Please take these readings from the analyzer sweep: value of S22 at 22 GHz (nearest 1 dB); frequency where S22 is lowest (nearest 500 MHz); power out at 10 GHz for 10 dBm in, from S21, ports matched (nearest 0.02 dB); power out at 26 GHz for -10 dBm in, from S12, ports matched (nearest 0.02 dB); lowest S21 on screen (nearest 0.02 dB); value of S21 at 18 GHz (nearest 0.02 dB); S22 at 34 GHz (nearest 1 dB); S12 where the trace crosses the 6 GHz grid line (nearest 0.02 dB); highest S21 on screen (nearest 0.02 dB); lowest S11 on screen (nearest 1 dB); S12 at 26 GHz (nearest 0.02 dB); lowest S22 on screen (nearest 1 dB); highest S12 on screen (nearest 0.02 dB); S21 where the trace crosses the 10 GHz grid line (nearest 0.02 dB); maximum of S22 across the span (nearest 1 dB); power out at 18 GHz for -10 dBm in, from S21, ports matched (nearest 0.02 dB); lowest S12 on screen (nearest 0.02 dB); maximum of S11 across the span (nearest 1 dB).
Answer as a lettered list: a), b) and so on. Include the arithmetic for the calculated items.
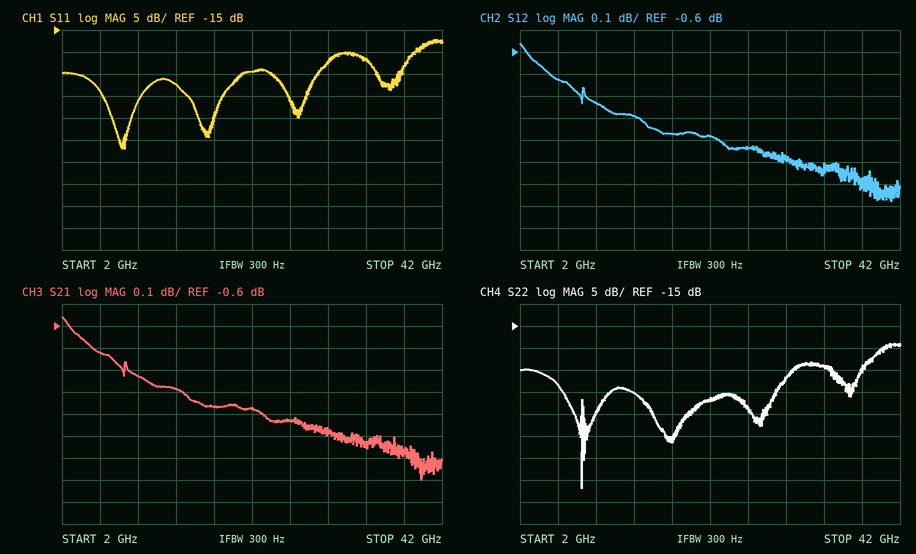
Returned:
a) -32 dB
b) 8.5 GHz
c) 10 dBm + (-0.82 dB) = 9.18 dBm
d) -10 dBm + (-1.04 dB) = -11.04 dBm
e) -1.30 dB
f) -0.96 dB
g) -24 dB
h) -0.72 dB
i) -0.56 dB
j) -42 dB
k) -1.04 dB
l) -52 dB
m) -0.56 dB
n) -0.82 dB
o) -19 dB
p) -10 dBm + (-0.96 dB) = -10.96 dBm
q) -1.28 dB
r) -17 dB
